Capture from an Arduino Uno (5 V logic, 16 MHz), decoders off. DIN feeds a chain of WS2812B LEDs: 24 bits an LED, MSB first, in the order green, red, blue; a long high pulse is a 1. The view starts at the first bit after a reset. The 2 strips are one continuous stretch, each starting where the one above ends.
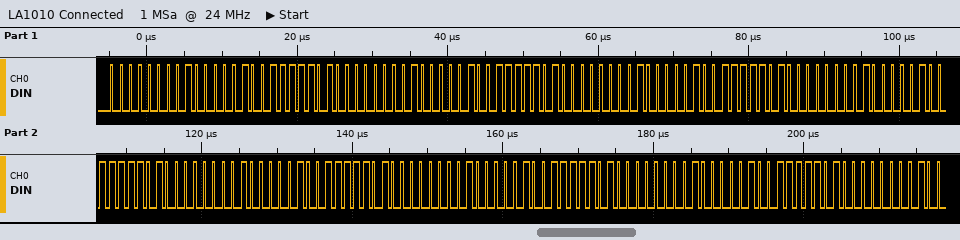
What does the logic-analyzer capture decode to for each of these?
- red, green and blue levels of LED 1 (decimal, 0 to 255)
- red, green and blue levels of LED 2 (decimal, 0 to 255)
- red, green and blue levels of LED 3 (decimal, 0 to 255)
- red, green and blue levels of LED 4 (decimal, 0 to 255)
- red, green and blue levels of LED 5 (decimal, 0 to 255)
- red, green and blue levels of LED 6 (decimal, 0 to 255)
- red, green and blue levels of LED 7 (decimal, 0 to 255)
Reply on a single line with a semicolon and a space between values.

130, 0, 125; 130, 0, 125; 130, 0, 125; 130, 0, 125; 130, 0, 125; 130, 0, 125; 130, 0, 125
